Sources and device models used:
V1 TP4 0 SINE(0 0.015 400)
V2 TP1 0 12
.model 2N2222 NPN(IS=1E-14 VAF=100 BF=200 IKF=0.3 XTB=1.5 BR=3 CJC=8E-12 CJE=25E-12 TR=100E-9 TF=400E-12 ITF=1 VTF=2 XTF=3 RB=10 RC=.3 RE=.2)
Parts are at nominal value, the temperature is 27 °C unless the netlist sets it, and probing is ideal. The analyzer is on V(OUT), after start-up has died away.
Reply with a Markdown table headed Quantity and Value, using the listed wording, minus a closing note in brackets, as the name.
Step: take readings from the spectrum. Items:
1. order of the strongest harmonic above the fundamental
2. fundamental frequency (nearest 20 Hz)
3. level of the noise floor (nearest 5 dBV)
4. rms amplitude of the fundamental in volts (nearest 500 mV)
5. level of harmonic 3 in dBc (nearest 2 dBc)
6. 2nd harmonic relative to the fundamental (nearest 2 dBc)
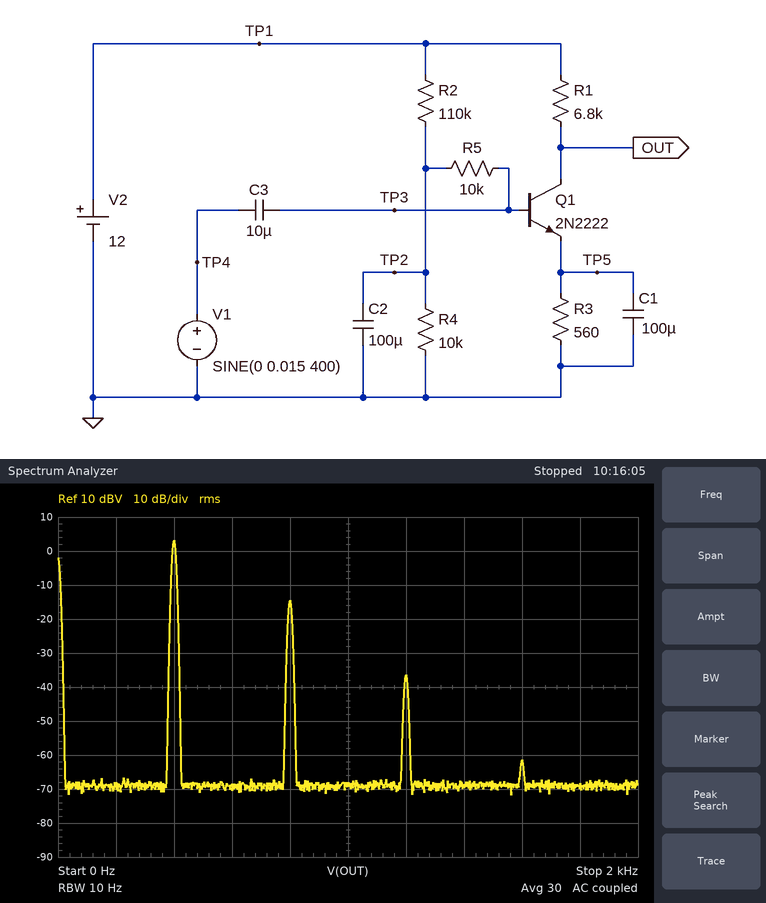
| Quantity | Value |
|---|---|
| order of the strongest harmonic above the fundamental | 2 |
| fundamental frequency | 400 Hz |
| level of the noise floor | -70 dBV |
| rms amplitude of the fundamental in volts | 1.5 V |
| level of harmonic 3 in dBc | -40 dBc |
| 2nd harmonic relative to the fundamental | -18 dBc |
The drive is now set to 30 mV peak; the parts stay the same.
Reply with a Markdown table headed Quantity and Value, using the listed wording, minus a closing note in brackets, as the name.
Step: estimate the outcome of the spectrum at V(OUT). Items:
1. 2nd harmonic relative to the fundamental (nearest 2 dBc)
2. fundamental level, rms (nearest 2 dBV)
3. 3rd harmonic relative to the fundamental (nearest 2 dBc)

| Quantity | Value |
|---|---|
| 2nd harmonic relative to the fundamental | -12 dBc |
| fundamental level, rms | 8 dBV |
| 3rd harmonic relative to the fundamental | -28 dBc |
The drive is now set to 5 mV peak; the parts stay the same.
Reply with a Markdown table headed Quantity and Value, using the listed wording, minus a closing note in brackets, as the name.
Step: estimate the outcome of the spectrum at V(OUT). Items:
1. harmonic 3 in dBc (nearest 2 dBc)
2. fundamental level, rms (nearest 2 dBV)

| Quantity | Value |
|---|---|
| harmonic 3 in dBc | -58 dBc |
| fundamental level, rms | -6 dBV |
